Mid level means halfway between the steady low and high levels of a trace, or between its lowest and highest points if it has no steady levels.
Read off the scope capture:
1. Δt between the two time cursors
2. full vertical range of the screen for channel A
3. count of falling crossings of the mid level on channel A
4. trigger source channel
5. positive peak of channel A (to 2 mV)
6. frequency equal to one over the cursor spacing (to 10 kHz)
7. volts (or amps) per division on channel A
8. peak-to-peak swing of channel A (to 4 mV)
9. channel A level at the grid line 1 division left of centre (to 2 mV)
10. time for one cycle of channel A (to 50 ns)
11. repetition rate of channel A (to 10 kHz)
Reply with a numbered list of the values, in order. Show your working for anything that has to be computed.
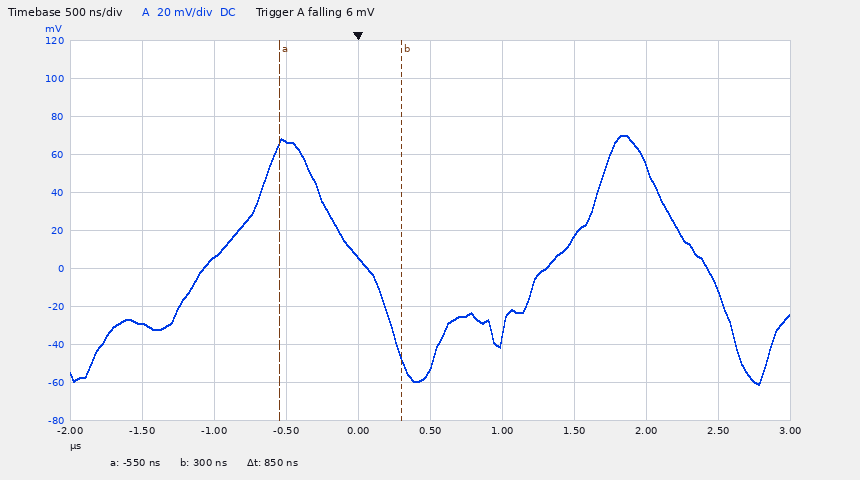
1. 850 ns
2. 200 mV
3. 2
4. channel A
5. 70 mV
6. 1 / 850 ns ≈ 1.18 MHz
7. 20 mV
8. 132 mV
9. 6 mV
10. 2.40 µs
11. 1 / 2.40 µs ≈ 417 kHz, so 420 kHz to the nearest 10 kHz
